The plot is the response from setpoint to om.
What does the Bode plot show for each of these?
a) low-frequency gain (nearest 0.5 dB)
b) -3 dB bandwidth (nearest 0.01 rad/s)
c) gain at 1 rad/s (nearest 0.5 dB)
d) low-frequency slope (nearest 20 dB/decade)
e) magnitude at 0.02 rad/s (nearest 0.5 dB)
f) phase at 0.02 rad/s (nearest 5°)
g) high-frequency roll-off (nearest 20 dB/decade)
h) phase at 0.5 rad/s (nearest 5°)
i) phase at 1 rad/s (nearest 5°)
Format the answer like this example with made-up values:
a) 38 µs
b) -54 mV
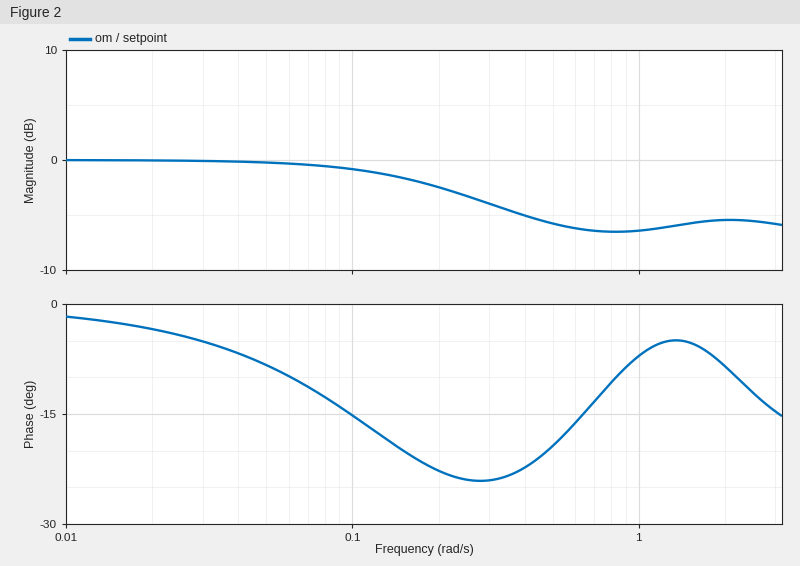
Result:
a) 0.0 dB
b) 0.23 rad/s
c) -6.5 dB
d) 0 dB/decade
e) 0.0 dB
f) -5°
g) 0 dB/decade
h) -20°
i) -5°
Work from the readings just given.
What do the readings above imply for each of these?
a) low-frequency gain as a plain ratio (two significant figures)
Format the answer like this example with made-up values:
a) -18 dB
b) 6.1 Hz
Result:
a) 1.0
